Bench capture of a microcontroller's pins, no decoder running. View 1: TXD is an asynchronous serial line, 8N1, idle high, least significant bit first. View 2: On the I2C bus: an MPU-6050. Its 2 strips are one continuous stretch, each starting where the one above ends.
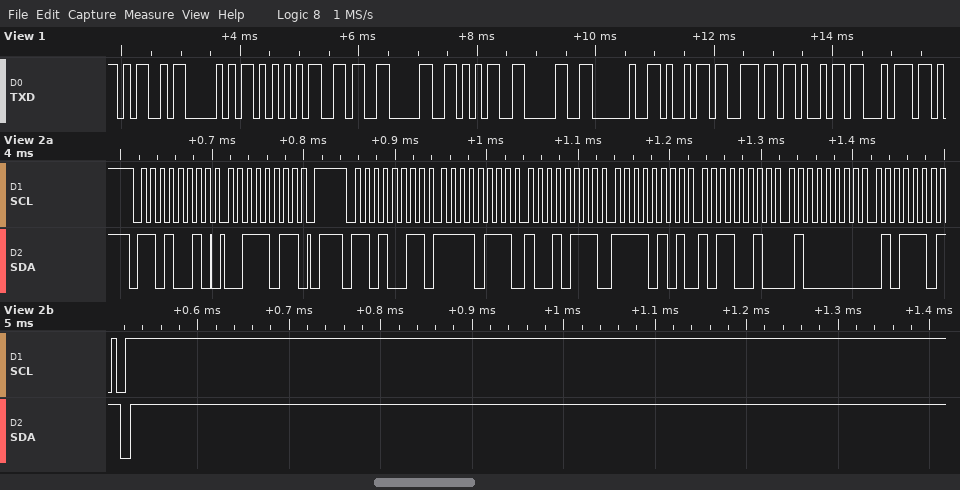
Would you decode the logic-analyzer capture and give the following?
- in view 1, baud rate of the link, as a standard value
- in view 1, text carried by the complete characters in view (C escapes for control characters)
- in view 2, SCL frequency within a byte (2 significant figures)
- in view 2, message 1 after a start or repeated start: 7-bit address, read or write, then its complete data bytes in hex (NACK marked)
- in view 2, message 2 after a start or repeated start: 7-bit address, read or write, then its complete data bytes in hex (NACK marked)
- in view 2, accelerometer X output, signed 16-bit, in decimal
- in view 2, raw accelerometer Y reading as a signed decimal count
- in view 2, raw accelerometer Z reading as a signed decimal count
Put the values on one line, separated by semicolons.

9600 baud; "MPU6050 init"; 100 kHz; 0x69 write: 3B; 0x69 read: F7 97 F5 B2 40 5D NACK; -2153; -2638; 16477
